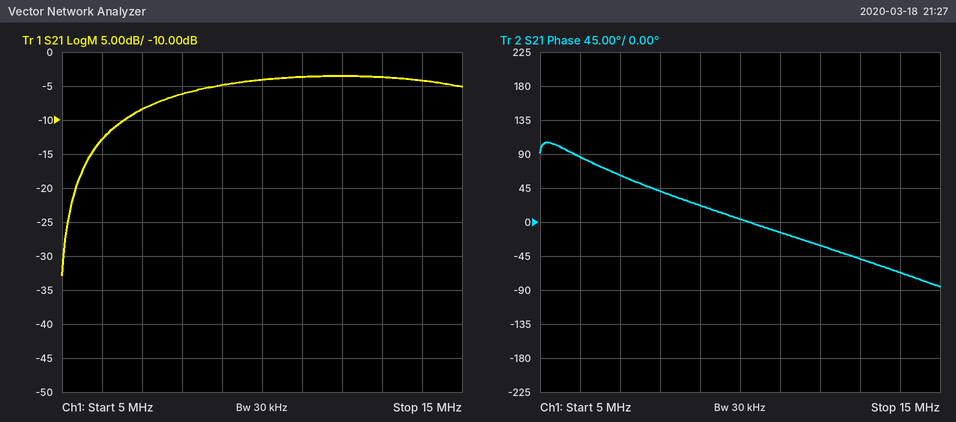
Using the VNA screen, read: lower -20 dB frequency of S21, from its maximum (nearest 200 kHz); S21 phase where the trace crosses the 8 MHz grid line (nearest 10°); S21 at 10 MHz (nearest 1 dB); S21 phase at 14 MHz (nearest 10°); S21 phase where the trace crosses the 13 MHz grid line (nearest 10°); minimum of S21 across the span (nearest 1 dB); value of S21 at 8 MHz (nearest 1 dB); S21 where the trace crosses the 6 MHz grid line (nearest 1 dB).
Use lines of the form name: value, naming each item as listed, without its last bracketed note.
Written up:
lower -20 dB frequency of S21, from its maximum: 5.2 MHz
S21 phase where the trace crosses the 8 MHz grid line: 40°
S21 at 10 MHz: -4 dB
S21 phase at 14 MHz: -70°
S21 phase where the trace crosses the 13 MHz grid line: -50°
minimum of S21 across the span: -33 dB
value of S21 at 8 MHz: -6 dB
S21 where the trace crosses the 6 MHz grid line: -13 dB
